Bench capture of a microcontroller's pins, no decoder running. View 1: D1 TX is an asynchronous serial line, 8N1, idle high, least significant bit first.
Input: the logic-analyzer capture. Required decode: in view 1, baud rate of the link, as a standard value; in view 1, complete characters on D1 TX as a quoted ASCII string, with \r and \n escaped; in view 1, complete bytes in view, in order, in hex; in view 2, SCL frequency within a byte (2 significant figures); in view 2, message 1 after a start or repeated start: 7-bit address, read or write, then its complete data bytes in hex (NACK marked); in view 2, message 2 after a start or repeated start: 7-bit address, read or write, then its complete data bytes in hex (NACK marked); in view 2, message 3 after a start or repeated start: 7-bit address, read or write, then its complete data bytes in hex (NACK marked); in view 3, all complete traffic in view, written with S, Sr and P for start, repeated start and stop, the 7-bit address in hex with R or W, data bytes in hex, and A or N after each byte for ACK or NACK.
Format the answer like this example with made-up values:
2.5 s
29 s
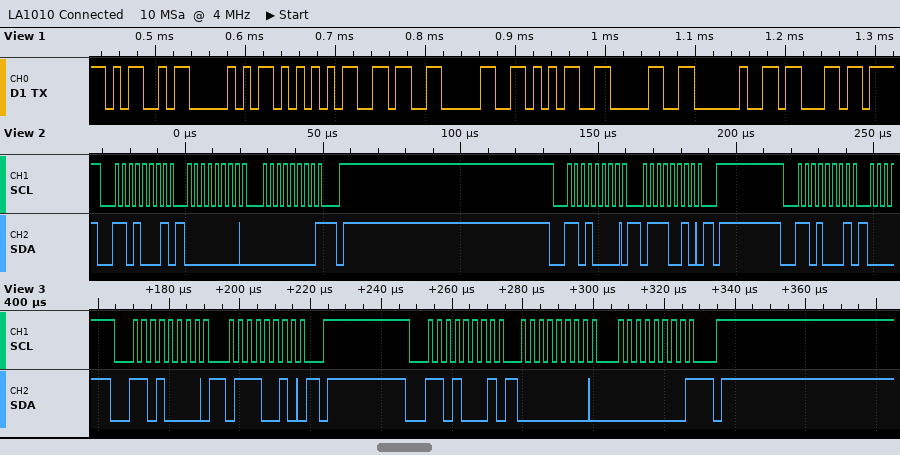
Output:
115200 baud
"MPU6050 c"
4D 50 55 36 30 35 30 20 63
400 kHz
0x68 read: 00 00 NACK
0x68 write: 72
0x68 read
S 68W A 72 A P S 68R A 00 A 00 N P
